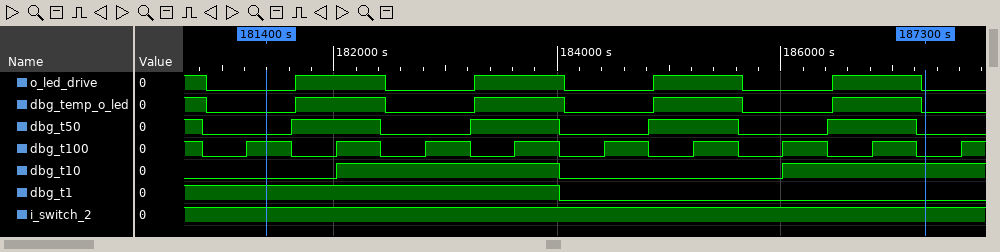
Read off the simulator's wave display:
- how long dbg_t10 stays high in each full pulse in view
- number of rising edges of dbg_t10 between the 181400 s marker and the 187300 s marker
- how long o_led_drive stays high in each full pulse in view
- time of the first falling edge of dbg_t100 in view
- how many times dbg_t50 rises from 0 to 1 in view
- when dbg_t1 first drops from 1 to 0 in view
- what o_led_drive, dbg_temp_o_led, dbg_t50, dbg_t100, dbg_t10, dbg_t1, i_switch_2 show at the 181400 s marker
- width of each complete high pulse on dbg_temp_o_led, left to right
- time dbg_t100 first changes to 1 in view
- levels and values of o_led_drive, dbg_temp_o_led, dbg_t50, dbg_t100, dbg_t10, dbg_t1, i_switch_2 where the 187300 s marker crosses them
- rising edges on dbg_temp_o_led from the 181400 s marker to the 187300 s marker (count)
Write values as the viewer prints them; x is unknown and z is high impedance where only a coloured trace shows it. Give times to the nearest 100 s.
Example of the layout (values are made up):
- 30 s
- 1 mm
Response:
- 2000 s
- 2
- 800 s, 800 s, 800 s, 800 s
- 180800 s
- 4
- 184000 s
- o_led_drive=0, dbg_temp_o_led=0, dbg_t50=0, dbg_t100=1, dbg_t10=0, dbg_t1=1, i_switch_2=1
- 800 s, 800 s, 800 s, 800 s
- 181200 s
- o_led_drive=0, dbg_temp_o_led=0, dbg_t50=0, dbg_t100=0, dbg_t10=1, dbg_t1=0, i_switch_2=1
- 4
